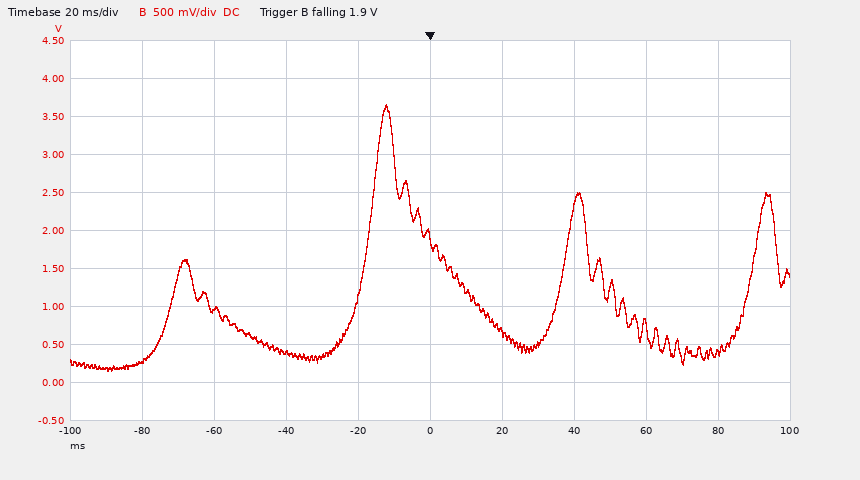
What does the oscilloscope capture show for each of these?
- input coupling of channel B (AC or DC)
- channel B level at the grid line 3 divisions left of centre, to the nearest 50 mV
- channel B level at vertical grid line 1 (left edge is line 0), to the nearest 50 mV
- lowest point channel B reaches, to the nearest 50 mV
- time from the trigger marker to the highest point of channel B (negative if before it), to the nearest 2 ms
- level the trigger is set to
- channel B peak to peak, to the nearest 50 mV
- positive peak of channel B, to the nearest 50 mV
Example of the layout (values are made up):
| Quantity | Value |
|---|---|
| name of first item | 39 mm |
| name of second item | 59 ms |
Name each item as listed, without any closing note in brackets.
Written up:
| Quantity | Value |
|---|---|
| input coupling of channel B | DC |
| channel B level at the grid line 3 divisions left of centre, to the nearest 50 mV | 950 mV |
| channel B level at vertical grid line 1 (left edge is line 0), to the nearest 50 mV | 300 mV |
| lowest point channel B reaches, to the nearest 50 mV | 150 mV |
| time from the trigger marker to the highest point of channel B (negative if before it), to the nearest 2 ms | -12 ms |
| level the trigger is set to | 1.9 V |
| channel B peak to peak, to the nearest 50 mV | 3.50 V |
| positive peak of channel B, to the nearest 50 mV | 3.65 V |
